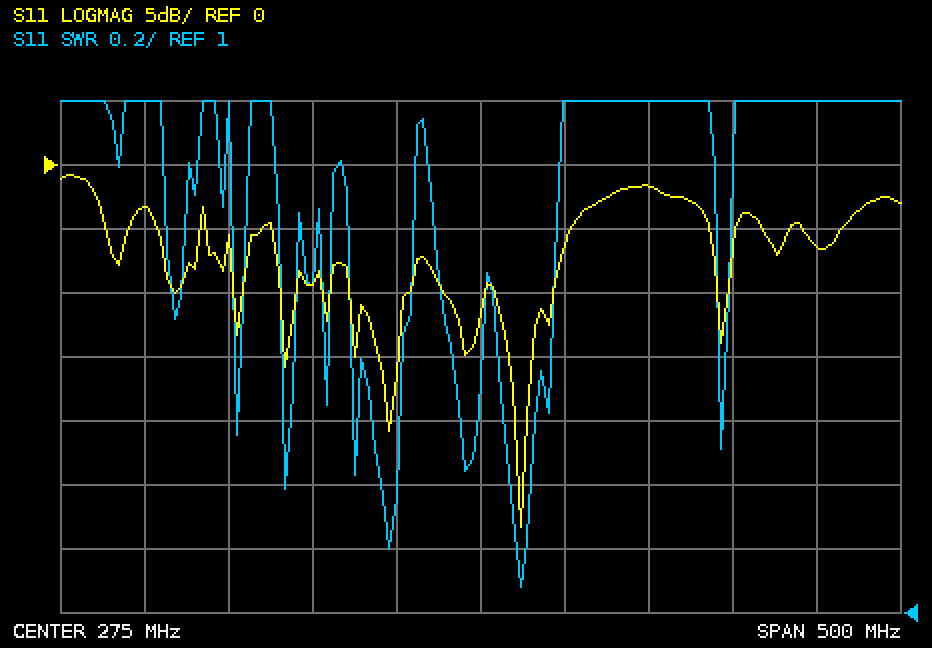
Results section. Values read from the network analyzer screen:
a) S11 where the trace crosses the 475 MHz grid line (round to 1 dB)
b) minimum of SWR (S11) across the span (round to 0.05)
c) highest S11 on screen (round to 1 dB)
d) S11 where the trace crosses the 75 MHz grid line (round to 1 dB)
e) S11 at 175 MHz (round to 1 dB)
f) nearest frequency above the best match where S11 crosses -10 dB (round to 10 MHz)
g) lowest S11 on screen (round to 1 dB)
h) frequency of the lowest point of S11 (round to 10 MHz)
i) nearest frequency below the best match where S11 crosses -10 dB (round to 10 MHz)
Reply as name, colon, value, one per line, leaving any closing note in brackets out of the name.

S11 where the trace crosses the 475 MHz grid line: -6 dB
minimum of SWR (S11) across the span: 1.10
highest S11 on screen: -1 dB
S11 where the trace crosses the 75 MHz grid line: -3 dB
S11 at 175 MHz: -9 dB
nearest frequency above the best match where S11 crosses -10 dB: 320 MHz
lowest S11 on screen: -28 dB
frequency of the lowest point of S11: 300 MHz
nearest frequency below the best match where S11 crosses -10 dB: 280 MHz
